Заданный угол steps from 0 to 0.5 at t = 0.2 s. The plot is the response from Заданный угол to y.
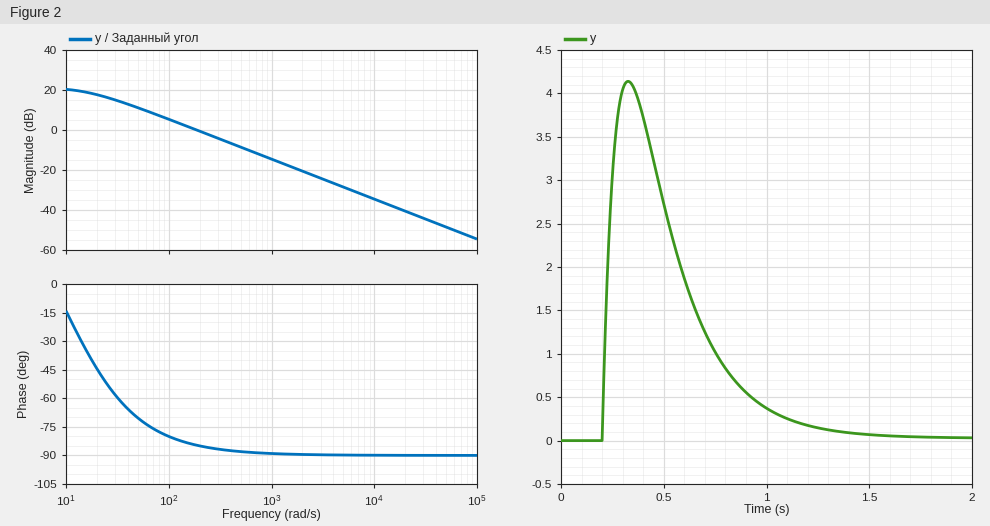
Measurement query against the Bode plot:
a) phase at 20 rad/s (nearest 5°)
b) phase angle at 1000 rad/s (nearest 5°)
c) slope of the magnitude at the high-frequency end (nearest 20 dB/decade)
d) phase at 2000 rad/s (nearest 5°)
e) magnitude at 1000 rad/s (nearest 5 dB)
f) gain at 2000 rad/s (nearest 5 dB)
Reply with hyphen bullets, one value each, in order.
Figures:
- -45°
- -90°
- -20 dB/decade
- -90°
- -15 dB
- -20 dB
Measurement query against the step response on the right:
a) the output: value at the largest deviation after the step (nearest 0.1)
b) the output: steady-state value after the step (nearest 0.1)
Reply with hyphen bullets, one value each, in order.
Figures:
- 4.1
- 0.0
